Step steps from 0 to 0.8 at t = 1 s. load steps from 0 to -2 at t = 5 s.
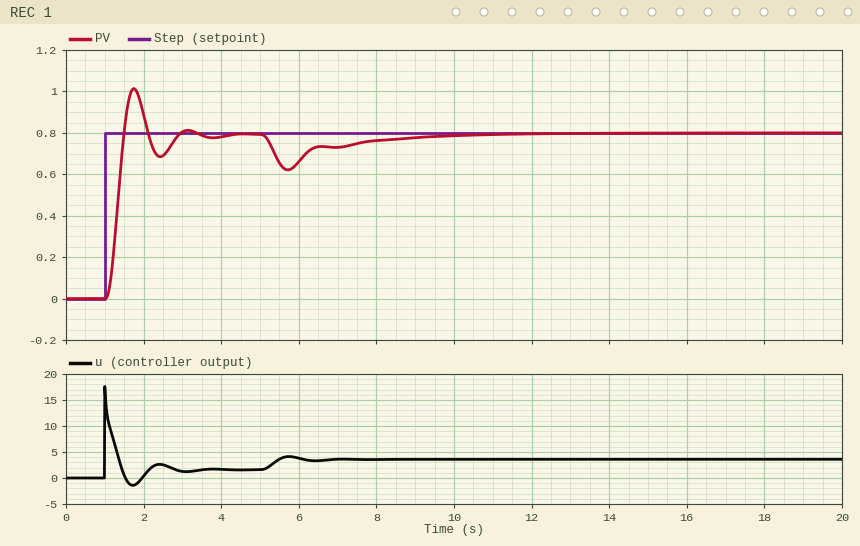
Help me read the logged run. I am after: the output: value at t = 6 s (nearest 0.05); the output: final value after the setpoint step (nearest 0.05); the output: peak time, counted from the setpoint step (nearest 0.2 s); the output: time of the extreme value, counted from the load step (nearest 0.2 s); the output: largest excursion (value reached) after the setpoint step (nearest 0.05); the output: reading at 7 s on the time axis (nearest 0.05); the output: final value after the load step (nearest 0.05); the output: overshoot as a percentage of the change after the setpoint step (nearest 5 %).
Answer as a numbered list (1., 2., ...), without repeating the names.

1. 0.65
2. 0.80
3. 0.8 s
4. 0.8 s
5. 1.00
6. 0.75
7. 0.80
8. 25 %
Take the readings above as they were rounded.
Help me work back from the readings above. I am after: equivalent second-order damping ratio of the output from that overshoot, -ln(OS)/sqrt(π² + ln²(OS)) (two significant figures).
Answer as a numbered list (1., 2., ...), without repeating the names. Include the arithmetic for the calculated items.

1. ln(0.25) = -1.386; 1.386 / sqrt(9.870 + 1.922) = 0.40
